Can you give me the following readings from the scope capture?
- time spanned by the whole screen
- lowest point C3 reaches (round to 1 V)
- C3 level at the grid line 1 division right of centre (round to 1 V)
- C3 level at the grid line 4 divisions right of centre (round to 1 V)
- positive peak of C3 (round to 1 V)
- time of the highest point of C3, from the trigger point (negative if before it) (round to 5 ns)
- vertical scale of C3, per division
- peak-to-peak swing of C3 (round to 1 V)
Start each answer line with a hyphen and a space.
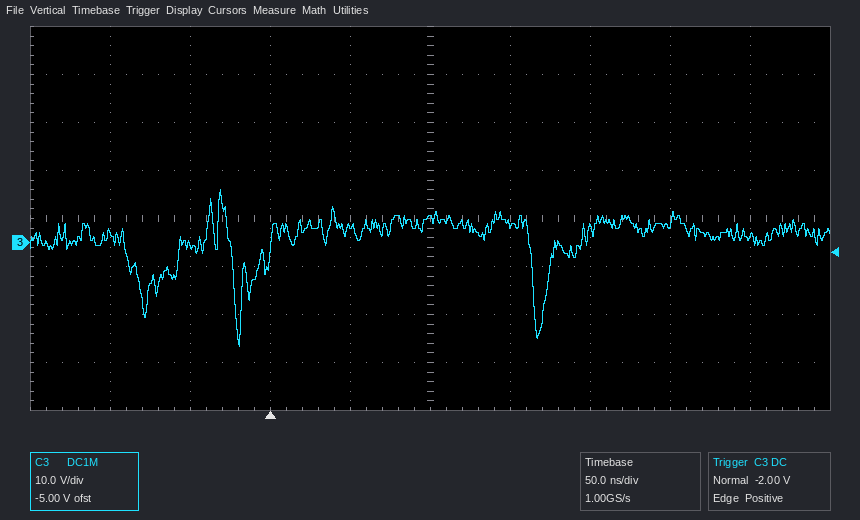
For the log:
- 500 ns
- -22 V
- 4 V
- 1 V
- 11 V
- -30 ns
- 10 V
- 33 V
